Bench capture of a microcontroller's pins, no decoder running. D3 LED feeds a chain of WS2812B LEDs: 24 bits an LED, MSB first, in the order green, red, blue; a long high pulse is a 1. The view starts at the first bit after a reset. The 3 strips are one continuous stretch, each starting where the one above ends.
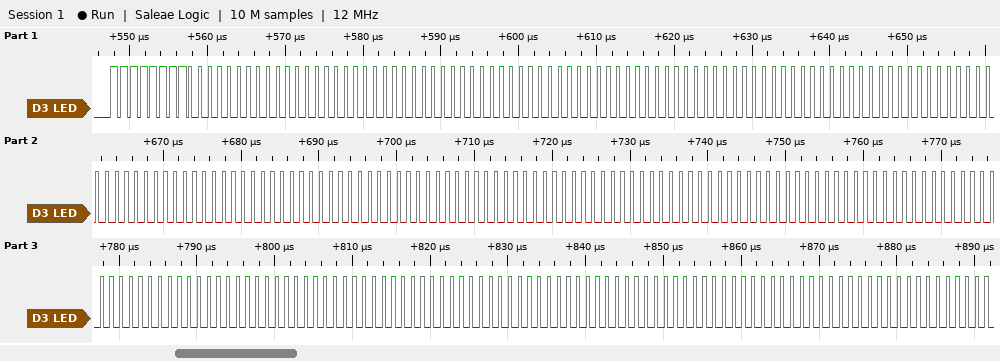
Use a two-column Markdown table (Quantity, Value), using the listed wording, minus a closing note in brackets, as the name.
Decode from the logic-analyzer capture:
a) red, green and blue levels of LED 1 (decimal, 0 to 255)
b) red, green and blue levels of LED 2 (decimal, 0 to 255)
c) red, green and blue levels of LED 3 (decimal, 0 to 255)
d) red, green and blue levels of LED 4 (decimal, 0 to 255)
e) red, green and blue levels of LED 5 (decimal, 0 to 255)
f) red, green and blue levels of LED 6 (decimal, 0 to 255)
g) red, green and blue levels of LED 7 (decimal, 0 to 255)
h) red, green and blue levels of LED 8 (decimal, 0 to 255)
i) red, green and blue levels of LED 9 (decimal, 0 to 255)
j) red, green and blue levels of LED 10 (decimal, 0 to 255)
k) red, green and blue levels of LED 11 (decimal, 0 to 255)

| Quantity | Value |
|---|---|
| red, green and blue levels of LED 1 | 0, 255, 0 |
| red, green and blue levels of LED 2 | 0, 0, 0 |
| red, green and blue levels of LED 3 | 0, 0, 0 |
| red, green and blue levels of LED 4 | 0, 0, 0 |
| red, green and blue levels of LED 5 | 0, 0, 0 |
| red, green and blue levels of LED 6 | 0, 0, 0 |
| red, green and blue levels of LED 7 | 0, 0, 0 |
| red, green and blue levels of LED 8 | 0, 0, 0 |
| red, green and blue levels of LED 9 | 0, 0, 0 |
| red, green and blue levels of LED 10 | 0, 0, 0 |
| red, green and blue levels of LED 11 | 0, 0, 0 |
